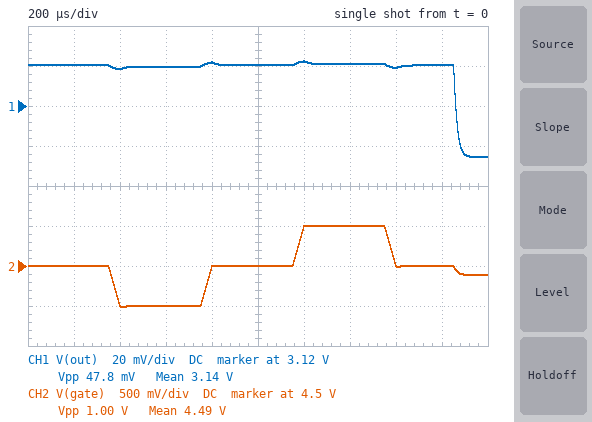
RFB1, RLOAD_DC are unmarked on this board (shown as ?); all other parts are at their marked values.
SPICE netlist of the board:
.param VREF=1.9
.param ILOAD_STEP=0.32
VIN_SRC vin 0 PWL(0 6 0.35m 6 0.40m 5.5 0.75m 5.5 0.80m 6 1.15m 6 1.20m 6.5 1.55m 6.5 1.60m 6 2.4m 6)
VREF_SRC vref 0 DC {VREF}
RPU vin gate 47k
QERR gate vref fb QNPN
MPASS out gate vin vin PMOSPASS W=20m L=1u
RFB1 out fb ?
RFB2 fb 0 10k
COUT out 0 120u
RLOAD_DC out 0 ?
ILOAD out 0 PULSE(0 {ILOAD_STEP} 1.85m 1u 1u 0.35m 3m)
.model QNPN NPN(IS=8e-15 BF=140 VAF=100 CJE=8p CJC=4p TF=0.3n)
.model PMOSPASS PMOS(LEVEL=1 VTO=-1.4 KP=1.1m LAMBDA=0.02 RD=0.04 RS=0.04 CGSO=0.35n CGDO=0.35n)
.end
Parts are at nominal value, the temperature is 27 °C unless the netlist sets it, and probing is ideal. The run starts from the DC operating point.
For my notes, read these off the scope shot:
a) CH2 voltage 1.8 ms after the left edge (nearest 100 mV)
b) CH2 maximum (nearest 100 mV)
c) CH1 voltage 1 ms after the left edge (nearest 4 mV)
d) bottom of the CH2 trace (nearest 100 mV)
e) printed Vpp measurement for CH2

4.5 V
5.0 V
3.140 V
4.0 V
1.00 V
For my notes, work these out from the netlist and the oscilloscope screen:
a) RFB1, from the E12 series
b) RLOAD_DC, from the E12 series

18 kΩ
27 Ω
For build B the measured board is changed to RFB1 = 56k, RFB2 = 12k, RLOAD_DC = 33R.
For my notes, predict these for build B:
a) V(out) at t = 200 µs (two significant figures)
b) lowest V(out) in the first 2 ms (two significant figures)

5.7 V
5.5 V
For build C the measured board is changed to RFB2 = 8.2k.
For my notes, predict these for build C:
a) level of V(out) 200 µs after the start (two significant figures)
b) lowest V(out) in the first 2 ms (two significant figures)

3.7 V
3.6 V
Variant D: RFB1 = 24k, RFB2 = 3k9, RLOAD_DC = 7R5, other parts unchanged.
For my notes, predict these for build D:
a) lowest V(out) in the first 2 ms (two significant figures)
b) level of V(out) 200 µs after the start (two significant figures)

5.4 V
5.9 V
